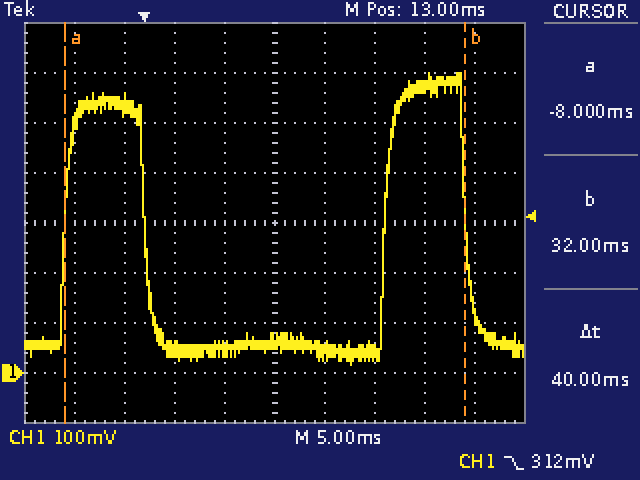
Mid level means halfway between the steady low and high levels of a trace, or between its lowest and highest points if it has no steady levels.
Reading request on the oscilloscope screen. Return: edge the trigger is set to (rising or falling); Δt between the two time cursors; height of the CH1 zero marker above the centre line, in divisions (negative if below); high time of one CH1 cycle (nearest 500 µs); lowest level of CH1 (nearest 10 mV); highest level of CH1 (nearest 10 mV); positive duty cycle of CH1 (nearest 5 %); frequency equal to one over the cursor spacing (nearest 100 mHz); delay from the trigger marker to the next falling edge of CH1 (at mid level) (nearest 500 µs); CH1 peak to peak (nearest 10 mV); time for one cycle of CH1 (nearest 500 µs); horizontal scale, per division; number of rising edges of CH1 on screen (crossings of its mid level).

falling
40 ms
-3.0 div
8.0 ms
20 mV
600 mV
25 %
25.0 Hz
32.0 ms
580 mV
32.0 ms
5 ms
2
